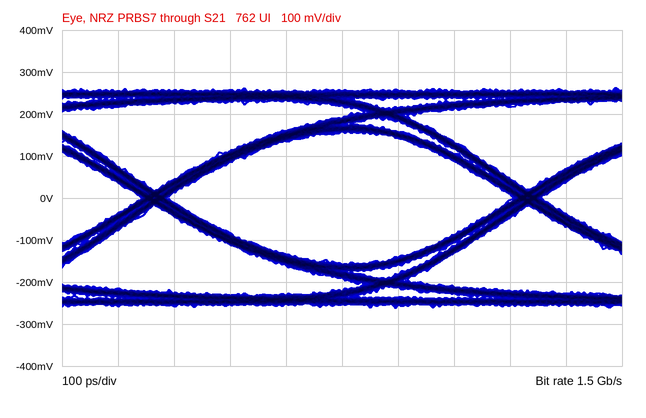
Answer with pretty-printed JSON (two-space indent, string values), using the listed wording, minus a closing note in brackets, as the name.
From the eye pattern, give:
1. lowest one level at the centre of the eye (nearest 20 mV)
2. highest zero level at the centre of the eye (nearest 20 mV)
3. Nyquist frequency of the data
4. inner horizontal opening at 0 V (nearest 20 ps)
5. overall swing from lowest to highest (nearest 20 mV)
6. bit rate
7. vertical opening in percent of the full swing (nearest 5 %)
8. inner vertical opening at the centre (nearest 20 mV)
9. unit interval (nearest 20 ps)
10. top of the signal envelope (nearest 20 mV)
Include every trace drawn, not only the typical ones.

{
  "lowest one level at the centre of the eye": "160 mV",
  "highest zero level at the centre of the eye": "-160 mV",
  "Nyquist frequency of the data": "750 MHz",
  "inner horizontal opening at 0 V": "620 ps",
  "overall swing from lowest to highest": "520 mV",
  "bit rate": "1.5 Gb/s",
  "vertical opening in percent of the full swing": "60 %",
  "inner vertical opening at the centre": "320 mV",
  "unit interval": "660 ps",
  "top of the signal envelope": "260 mV"
}
